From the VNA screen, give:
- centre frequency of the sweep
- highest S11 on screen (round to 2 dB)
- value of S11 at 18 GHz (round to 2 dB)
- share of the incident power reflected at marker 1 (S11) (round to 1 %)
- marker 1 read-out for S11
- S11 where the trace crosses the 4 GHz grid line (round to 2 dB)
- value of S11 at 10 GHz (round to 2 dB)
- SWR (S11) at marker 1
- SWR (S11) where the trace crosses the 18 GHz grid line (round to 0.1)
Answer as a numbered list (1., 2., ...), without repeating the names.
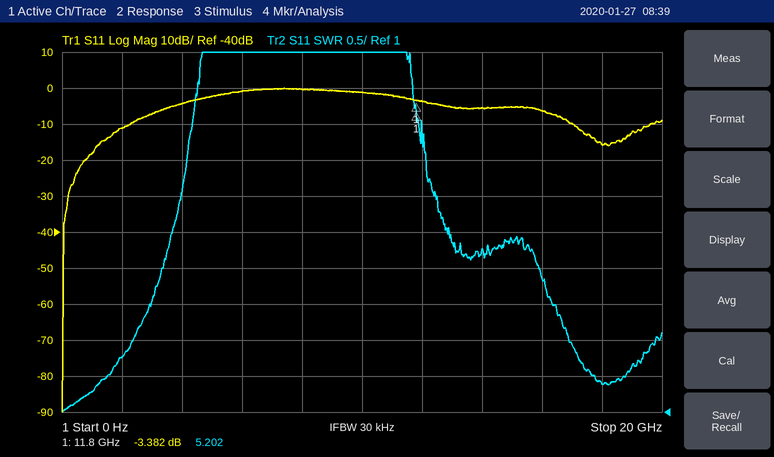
1. 10 GHz
2. 0 dB
3. -16 dB
4. 46 %
5. -3.382 dB
6. -4 dB
7. -2 dB
8. 5.202
9. 1.4
